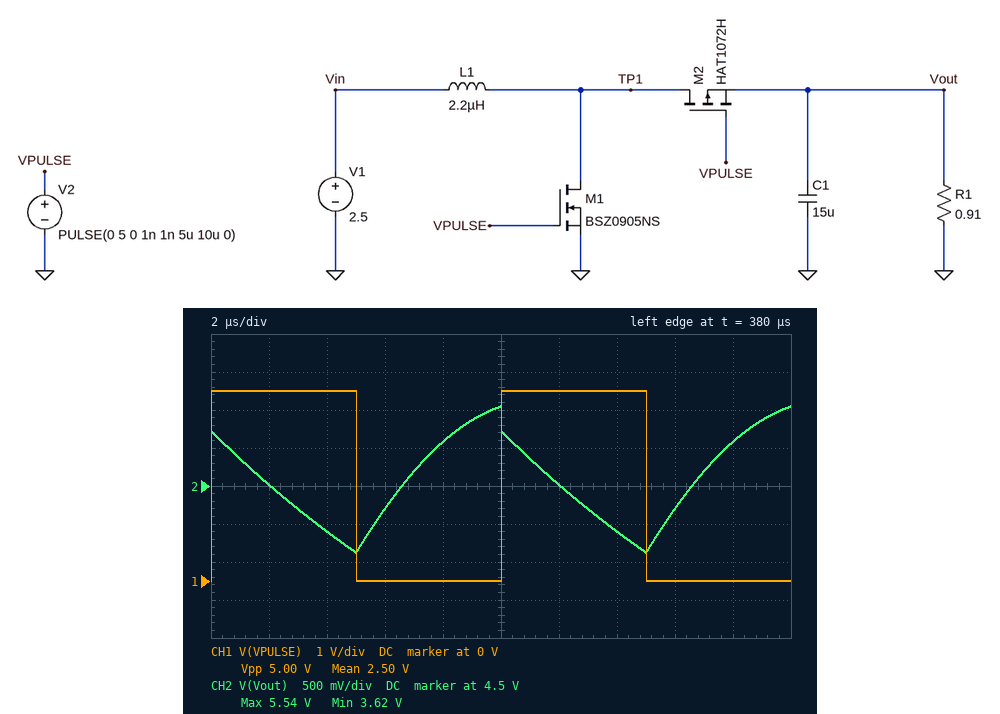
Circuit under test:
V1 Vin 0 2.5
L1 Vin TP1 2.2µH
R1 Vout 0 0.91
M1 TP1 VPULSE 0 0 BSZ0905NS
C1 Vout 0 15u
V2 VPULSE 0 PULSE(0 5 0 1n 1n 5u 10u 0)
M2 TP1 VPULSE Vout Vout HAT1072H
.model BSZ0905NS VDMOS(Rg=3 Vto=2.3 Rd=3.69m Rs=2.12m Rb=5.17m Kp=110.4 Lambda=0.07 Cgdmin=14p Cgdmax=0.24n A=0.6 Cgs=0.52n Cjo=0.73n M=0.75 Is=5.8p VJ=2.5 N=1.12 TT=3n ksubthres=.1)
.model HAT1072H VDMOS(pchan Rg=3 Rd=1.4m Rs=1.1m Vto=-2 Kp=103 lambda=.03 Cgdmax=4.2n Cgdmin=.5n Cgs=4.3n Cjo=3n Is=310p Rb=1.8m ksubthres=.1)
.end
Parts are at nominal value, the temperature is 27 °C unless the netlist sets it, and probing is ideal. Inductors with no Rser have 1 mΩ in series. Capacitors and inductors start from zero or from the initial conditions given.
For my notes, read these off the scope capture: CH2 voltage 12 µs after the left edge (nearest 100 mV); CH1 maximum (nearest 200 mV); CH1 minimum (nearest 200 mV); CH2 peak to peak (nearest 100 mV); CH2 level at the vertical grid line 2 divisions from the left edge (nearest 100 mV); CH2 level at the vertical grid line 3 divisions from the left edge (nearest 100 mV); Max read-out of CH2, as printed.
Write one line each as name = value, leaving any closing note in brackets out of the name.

CH2 voltage 12 µs after the left edge = 4.5 V
CH1 maximum = 5.0 V
CH1 minimum = 0 V
CH2 peak to peak = 1.9 V
CH2 level at the vertical grid line 2 divisions from the left edge = 3.9 V
CH2 level at the vertical grid line 3 divisions from the left edge = 4.2 V
Max read-out of CH2, as printed = 5.54 V
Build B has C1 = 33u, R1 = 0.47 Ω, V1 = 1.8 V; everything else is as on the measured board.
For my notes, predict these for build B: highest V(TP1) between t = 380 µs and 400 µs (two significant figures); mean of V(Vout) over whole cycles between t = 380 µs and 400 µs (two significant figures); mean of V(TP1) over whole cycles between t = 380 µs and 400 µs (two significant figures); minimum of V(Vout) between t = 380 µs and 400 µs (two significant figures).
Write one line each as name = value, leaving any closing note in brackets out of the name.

highest V(TP1) between t = 380 µs and 400 µs = 3.9 V
mean of V(Vout) over whole cycles between t = 380 µs and 400 µs = 3.2 V
mean of V(TP1) over whole cycles between t = 380 µs and 400 µs = 1.8 V
minimum of V(Vout) between t = 380 µs and 400 µs = 2.7 V
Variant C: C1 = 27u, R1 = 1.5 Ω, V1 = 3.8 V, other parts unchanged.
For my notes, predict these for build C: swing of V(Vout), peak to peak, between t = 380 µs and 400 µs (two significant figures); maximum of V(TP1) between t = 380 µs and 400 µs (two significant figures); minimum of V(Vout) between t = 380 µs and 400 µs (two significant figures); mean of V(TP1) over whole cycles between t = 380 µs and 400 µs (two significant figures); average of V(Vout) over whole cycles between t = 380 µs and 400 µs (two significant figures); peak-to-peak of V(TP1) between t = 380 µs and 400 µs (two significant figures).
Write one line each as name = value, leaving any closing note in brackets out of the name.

swing of V(Vout), peak to peak, between t = 380 µs and 400 µs = 1.6 V
maximum of V(TP1) between t = 380 µs and 400 µs = 8.0 V
minimum of V(Vout) between t = 380 µs and 400 µs = 6.4 V
mean of V(TP1) over whole cycles between t = 380 µs and 400 µs = 3.8 V
average of V(Vout) over whole cycles between t = 380 µs and 400 µs = 7.1 V
peak-to-peak of V(TP1) between t = 380 µs and 400 µs = 7.9 V
